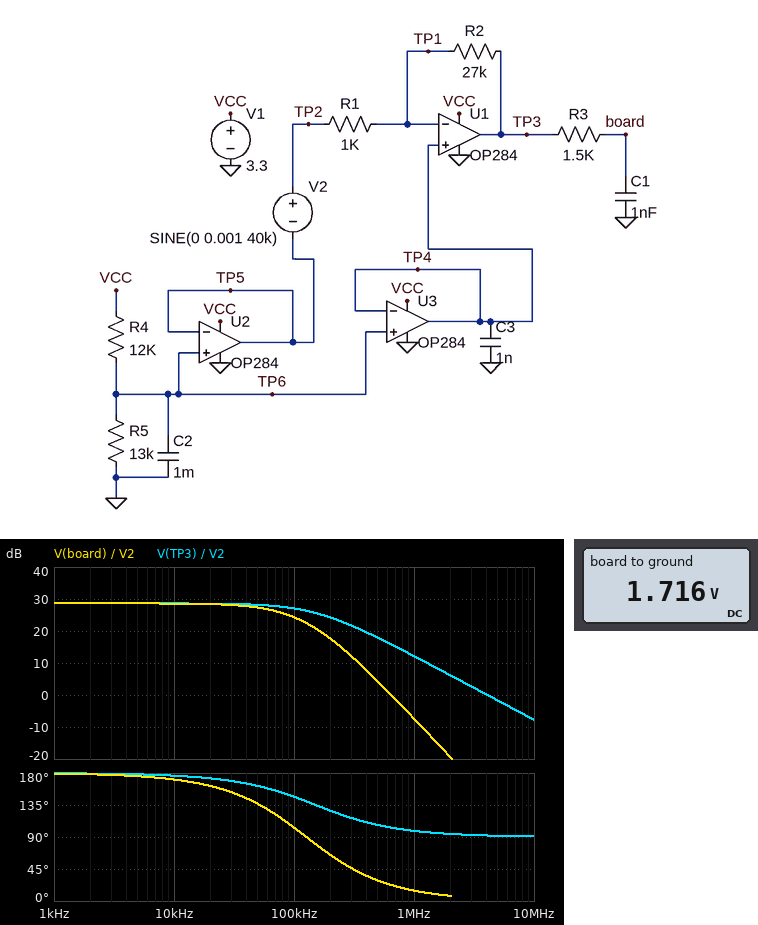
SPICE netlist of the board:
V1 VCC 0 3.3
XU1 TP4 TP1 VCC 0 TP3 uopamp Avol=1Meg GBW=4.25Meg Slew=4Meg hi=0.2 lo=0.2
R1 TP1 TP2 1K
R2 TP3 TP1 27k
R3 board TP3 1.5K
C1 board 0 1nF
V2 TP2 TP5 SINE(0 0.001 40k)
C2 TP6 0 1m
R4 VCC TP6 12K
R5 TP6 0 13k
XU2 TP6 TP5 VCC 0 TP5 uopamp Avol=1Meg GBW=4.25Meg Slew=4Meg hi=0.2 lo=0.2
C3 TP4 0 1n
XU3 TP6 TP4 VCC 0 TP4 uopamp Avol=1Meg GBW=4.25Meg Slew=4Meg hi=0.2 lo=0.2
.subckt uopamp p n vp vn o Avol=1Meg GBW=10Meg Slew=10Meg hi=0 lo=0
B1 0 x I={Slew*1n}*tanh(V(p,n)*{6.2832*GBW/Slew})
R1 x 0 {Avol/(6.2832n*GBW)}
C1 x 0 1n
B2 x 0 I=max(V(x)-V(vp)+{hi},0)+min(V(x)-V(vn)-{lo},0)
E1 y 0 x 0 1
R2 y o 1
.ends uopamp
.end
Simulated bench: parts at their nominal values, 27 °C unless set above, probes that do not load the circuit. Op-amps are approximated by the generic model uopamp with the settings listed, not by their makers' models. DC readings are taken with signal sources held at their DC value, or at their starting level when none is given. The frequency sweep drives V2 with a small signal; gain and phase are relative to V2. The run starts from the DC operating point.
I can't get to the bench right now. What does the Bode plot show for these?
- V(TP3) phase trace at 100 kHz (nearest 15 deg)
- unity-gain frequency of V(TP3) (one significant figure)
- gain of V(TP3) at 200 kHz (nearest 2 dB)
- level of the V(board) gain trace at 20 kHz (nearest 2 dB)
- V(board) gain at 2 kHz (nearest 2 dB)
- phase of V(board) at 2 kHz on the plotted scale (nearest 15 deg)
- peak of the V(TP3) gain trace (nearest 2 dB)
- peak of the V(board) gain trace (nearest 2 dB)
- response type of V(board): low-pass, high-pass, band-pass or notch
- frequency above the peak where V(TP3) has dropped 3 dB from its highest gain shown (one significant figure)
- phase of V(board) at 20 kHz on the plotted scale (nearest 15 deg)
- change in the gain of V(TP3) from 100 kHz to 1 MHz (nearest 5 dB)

150 deg
4 MHz
24 dB
28 dB
28 dB
180 deg
28 dB
28 dB
low-pass
200 kHz
165 deg
-15 dB
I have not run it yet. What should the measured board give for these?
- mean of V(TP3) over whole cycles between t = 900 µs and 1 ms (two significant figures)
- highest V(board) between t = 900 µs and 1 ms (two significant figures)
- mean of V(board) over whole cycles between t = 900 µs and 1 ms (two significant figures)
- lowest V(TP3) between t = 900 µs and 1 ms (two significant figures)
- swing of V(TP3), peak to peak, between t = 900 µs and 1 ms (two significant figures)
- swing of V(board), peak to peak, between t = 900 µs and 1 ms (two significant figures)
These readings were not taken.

1.7 V
1.7 V
1.7 V
1.7 V
52 mV
49 mV
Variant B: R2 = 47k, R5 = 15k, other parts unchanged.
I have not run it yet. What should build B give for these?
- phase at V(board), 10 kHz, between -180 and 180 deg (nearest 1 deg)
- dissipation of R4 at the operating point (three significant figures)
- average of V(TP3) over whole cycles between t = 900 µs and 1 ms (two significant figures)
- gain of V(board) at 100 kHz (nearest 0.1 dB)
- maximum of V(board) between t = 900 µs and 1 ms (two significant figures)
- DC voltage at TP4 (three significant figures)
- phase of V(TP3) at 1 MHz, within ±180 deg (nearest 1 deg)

168 deg
179 µW
1.8 V
27.1 dB
1.9 V
1.83 V
95 deg
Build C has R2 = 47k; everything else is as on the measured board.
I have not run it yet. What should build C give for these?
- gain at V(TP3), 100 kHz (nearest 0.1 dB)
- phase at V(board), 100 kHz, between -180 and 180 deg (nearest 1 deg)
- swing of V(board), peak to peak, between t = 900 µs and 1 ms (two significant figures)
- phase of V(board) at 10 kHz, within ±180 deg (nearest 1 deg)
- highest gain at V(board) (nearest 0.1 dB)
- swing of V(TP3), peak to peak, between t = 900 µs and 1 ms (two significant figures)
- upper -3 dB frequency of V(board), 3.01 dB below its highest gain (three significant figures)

29.9 dB
88 deg
80 mV
168 deg
33.4 dB
86 mV
62.0 kHz
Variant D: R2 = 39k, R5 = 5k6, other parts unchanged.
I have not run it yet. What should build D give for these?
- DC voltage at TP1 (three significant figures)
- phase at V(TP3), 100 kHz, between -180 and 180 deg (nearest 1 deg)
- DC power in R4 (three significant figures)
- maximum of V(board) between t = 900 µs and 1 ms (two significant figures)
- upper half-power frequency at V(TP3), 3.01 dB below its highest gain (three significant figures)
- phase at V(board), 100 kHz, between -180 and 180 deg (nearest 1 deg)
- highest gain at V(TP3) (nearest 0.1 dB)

1.05 V
137 deg
422 µW
1.1 V
106 kHz
93 deg
31.8 dB
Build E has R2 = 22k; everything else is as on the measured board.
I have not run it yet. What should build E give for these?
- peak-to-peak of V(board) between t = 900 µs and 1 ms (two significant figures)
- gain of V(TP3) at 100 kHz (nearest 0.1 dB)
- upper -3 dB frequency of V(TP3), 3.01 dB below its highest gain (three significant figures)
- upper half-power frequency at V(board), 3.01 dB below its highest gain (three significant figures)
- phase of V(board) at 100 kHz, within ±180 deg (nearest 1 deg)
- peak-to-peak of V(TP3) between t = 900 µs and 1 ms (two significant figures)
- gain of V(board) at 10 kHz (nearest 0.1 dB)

40 mV
25.7 dB
185 kHz
85.4 kHz
108 deg
43 mV
26.8 dB
